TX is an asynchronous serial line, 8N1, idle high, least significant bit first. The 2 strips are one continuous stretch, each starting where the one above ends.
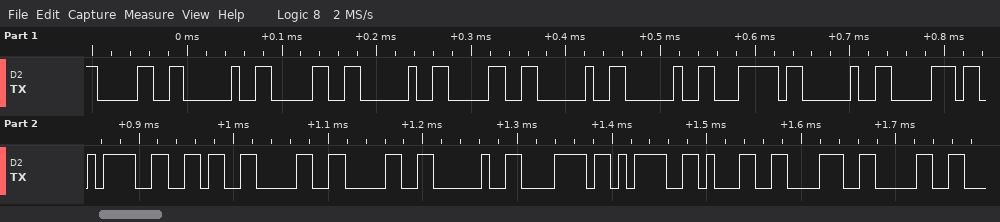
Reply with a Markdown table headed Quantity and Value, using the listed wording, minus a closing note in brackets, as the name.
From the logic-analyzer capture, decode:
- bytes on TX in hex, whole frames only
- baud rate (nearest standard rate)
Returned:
| Quantity | Value |
|---|---|
| bytes on TX in hex, whole frames only | 0x30 0x20 0x30 0x20 0x30 0x20 0x20 0x7C 0x20 0x70 0x3D 0x36 0x30 0x30 0x20 0x78 0x3D 0x31 0x38 0x30 |
| baud rate | 115200 baud |
